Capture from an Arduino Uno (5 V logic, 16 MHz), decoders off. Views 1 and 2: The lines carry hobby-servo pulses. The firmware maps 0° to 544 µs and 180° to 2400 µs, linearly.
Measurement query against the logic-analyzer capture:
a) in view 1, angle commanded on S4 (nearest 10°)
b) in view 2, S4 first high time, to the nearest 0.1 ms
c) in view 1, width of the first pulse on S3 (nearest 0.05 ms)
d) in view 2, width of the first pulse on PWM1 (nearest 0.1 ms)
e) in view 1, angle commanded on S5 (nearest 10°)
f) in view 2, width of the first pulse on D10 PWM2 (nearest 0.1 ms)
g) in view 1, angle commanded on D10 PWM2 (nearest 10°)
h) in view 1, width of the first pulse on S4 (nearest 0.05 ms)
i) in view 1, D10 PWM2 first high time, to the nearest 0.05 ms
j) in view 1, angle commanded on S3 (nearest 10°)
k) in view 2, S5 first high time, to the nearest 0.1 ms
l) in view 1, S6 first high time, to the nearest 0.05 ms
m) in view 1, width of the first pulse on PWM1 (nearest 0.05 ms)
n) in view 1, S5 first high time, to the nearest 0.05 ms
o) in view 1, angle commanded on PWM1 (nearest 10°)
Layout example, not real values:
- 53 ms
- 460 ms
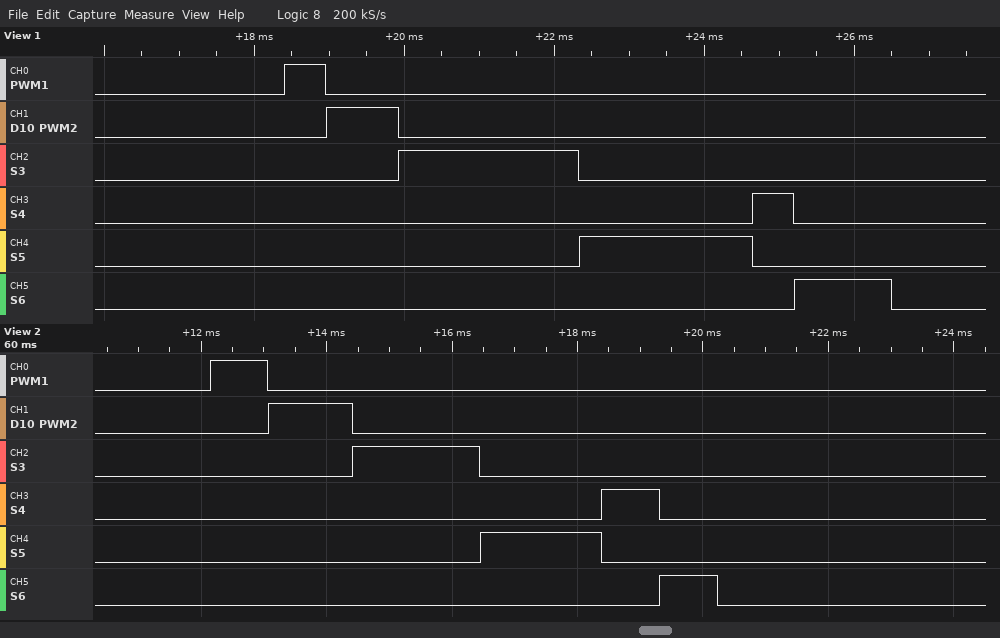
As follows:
- 0°
- 0.9 ms
- 2.40 ms
- 0.9 ms
- 170°
- 1.3 ms
- 40°
- 0.55 ms
- 0.95 ms
- 180°
- 1.9 ms
- 1.30 ms
- 0.55 ms
- 2.30 ms
- 0°
